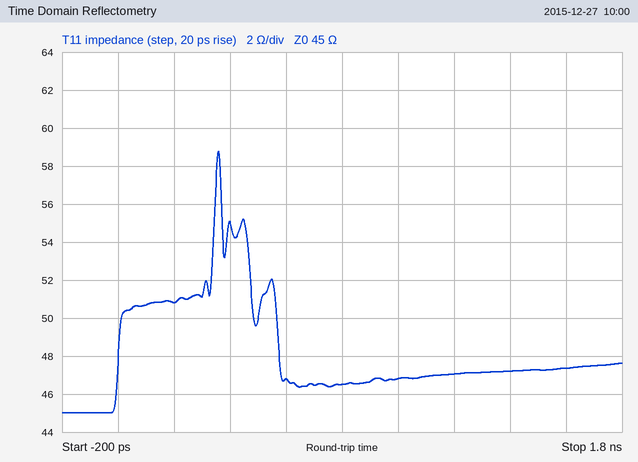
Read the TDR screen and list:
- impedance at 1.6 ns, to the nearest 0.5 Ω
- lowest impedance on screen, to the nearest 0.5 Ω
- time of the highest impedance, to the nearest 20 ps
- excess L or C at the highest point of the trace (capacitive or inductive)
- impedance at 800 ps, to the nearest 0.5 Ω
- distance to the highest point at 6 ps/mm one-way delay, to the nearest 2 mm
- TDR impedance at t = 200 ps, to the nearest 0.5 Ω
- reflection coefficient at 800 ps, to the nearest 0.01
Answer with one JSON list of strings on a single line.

["47.5 Ω", "45.0 Ω", "360 ps", "inductive", "46.5 Ω", "30 mm", "51.0 Ω", "+0.02"]
